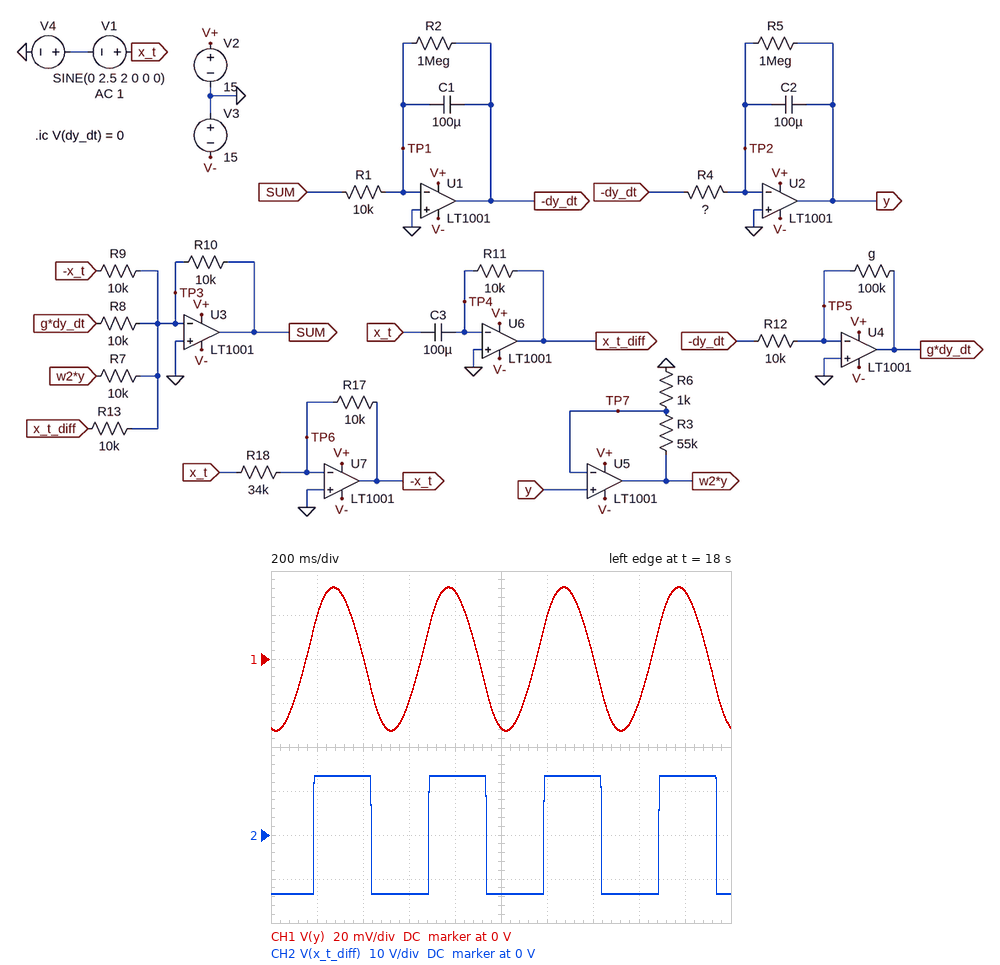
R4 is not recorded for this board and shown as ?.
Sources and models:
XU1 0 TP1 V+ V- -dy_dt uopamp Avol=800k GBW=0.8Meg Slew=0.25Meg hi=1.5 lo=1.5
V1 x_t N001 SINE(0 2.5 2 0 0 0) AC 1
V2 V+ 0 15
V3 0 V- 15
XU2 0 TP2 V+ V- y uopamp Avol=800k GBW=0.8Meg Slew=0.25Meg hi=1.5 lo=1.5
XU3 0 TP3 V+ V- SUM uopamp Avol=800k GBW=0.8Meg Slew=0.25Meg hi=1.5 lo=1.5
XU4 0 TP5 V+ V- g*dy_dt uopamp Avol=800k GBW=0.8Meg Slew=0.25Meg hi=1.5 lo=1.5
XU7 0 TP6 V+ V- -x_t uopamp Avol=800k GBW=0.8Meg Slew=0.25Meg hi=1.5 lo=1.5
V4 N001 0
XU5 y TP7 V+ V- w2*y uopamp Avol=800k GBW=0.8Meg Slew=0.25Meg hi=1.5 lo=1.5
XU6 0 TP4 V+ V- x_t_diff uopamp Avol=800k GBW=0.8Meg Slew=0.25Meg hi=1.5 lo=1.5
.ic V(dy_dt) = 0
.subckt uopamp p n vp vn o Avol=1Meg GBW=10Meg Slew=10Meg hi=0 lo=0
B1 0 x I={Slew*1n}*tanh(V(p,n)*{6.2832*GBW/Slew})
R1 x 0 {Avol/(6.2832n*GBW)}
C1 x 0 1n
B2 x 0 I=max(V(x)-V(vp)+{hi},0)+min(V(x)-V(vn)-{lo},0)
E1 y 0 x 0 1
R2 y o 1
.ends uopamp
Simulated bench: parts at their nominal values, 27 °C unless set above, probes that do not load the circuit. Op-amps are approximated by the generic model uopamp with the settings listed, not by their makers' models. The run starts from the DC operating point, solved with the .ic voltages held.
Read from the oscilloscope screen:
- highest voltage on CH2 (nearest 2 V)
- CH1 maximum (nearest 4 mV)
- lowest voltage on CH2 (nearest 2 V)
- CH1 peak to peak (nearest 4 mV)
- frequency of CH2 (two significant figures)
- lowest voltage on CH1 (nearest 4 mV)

14 V
32 mV
-14 V
64 mV
2.0 Hz
-32 mV
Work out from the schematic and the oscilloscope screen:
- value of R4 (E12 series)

27 kΩ
